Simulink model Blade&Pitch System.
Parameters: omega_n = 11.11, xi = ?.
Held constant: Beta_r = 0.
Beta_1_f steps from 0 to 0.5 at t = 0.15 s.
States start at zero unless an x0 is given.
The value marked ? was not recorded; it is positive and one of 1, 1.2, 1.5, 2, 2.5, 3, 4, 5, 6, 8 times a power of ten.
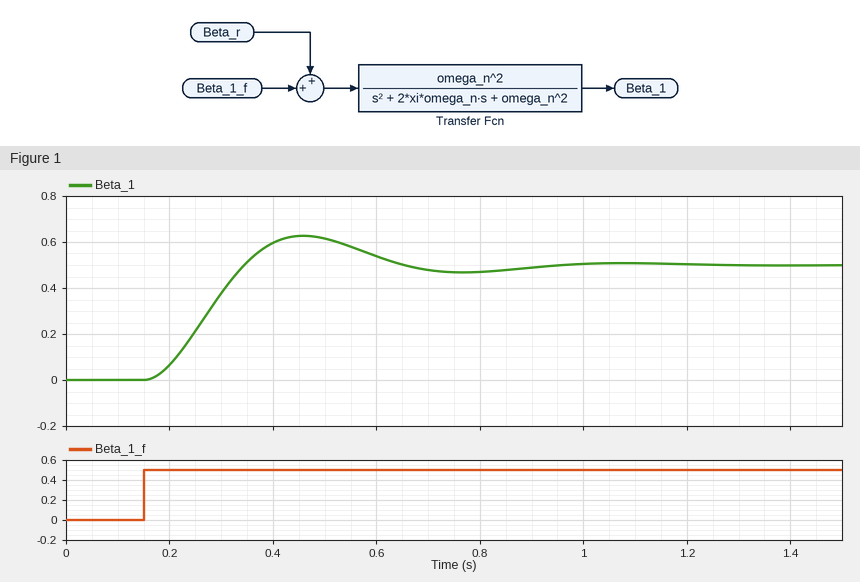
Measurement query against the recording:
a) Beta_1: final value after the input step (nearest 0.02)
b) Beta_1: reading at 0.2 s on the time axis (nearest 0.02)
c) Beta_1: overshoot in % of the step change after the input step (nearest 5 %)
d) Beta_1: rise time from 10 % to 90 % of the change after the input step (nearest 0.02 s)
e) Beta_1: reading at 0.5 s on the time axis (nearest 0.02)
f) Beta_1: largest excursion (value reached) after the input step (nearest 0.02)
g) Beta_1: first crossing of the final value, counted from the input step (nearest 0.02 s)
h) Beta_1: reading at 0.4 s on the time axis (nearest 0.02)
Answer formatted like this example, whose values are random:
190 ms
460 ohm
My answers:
0.50
0.06
25 %
0.14 s
0.62
0.62
0.20 s
0.60
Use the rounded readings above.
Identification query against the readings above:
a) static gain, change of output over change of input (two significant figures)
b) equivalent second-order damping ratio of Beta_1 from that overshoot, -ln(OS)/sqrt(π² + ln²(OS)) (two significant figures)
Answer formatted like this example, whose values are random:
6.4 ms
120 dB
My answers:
1.0
0.40
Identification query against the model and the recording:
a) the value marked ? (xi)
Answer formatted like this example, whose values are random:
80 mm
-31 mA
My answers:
0.4
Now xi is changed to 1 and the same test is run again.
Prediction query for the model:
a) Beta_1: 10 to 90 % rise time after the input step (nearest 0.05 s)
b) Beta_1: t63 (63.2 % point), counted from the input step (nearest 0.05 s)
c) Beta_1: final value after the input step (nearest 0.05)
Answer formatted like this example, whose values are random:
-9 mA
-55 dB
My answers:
0.30 s
0.20 s
0.50
